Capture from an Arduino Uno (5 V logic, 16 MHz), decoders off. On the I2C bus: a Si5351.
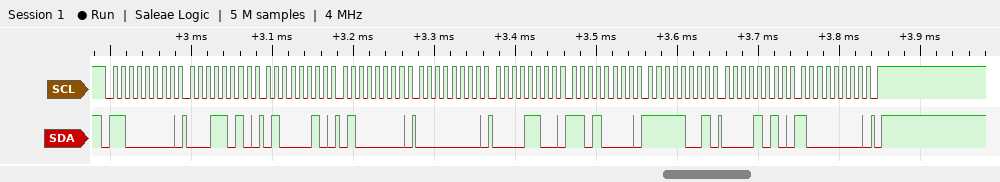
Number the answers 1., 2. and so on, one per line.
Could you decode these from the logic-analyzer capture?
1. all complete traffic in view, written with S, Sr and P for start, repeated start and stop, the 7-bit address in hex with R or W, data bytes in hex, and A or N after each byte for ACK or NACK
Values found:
1. S 60W A 1A A 42 A 40 A 00 A 0C A D0 A F9 A 0A A 80 A P
